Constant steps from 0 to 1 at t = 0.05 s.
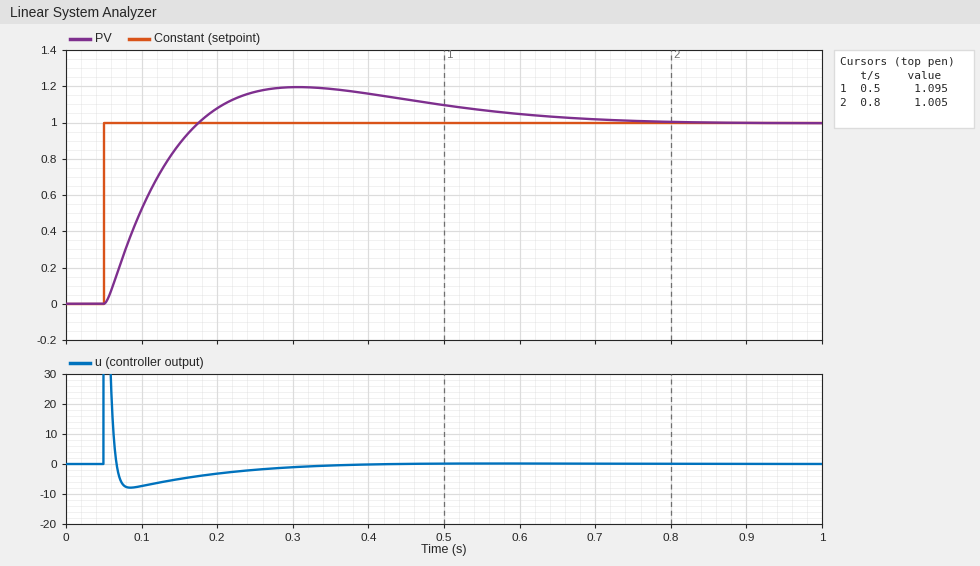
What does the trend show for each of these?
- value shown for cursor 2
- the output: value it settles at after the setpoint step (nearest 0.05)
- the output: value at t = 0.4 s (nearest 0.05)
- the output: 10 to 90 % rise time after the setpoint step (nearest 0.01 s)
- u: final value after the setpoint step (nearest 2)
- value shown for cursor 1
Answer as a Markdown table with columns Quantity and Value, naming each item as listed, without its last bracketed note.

| Quantity | Value |
|---|---|
| value shown for cursor 2 | 1.005 |
| the output: value it settles at after the setpoint step | 1.00 |
| the output: value at t = 0.4 s | 1.15 |
| the output: 10 to 90 % rise time after the setpoint step | 0.09 s |
| u: final value after the setpoint step | 0 |
| value shown for cursor 1 | 1.095 |
